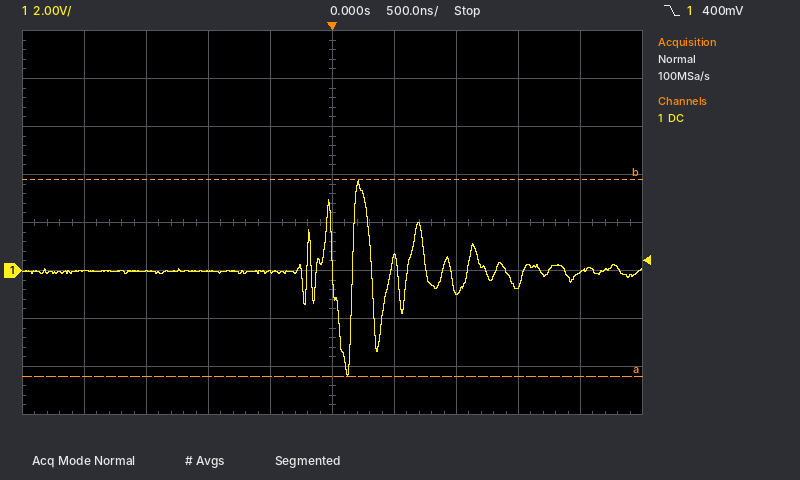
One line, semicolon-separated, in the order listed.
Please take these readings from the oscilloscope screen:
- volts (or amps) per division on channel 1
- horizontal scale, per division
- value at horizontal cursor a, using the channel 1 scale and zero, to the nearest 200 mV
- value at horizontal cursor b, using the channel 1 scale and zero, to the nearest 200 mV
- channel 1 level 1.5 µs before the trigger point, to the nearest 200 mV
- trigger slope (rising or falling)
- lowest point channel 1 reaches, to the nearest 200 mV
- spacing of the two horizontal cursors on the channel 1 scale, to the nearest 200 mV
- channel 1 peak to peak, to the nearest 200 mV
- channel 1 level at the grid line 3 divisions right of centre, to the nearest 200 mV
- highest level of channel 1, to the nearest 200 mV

2 V; 500 ns; -4.4 V; 3.8 V; 0.0 V; falling; -4.4 V; 8.2 V; 8.2 V; -600 mV; 3.8 V
